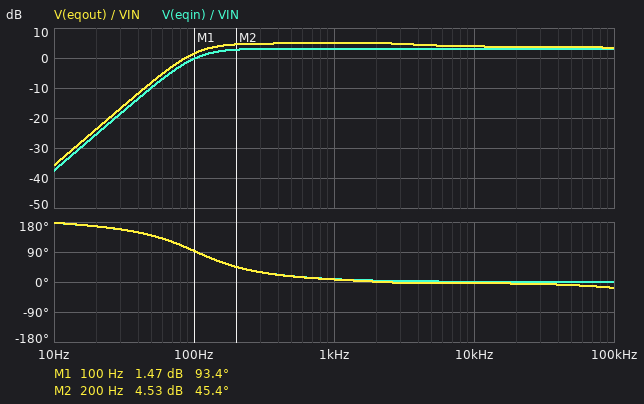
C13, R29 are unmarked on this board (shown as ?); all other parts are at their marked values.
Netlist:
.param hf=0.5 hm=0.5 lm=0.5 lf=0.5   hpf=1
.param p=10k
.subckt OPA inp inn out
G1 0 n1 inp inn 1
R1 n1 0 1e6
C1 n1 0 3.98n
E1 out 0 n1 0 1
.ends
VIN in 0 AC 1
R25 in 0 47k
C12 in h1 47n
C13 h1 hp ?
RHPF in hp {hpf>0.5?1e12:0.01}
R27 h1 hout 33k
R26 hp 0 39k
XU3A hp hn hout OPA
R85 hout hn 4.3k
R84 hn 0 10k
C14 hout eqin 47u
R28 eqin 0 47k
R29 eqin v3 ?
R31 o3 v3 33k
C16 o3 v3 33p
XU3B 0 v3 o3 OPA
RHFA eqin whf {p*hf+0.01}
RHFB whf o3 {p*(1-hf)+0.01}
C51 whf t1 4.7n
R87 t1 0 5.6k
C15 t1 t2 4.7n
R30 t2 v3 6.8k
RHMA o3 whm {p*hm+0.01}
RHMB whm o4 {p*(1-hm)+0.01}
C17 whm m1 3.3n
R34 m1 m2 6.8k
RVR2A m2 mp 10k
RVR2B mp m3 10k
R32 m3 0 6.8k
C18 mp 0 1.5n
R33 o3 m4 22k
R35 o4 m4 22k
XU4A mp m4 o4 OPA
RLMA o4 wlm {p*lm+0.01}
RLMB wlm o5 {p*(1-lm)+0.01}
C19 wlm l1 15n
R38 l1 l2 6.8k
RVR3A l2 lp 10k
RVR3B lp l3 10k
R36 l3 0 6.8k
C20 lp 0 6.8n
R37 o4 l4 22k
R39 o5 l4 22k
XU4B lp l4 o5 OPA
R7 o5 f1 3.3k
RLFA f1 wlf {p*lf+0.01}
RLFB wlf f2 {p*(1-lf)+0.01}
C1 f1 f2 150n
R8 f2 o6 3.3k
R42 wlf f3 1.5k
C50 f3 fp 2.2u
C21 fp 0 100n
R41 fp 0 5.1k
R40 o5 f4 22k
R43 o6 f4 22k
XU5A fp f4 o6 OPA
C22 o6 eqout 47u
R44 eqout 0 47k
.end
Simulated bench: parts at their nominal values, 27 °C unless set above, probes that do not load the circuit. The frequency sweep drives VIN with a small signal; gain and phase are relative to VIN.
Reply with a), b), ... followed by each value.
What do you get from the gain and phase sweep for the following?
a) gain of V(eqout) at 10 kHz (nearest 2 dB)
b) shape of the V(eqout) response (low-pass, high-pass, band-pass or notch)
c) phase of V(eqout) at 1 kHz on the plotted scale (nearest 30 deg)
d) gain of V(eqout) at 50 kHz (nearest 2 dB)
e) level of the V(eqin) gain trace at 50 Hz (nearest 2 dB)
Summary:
a) 4 dB
b) high-pass
c) 0 deg
d) 4 dB
e) -10 dB
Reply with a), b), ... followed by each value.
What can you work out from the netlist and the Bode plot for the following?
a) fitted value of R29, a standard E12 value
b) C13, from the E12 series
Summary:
a) 27 kΩ
b) 39 nF
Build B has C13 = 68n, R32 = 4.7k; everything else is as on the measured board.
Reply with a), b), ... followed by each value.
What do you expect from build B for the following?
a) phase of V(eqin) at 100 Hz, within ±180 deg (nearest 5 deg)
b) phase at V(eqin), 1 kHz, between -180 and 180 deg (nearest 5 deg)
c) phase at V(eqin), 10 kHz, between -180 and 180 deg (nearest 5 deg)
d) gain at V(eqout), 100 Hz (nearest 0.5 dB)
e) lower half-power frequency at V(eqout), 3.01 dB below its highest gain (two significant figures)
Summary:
a) 70 deg
b) 5 deg
c) 0 deg
d) 4.0 dB
e) 74 Hz
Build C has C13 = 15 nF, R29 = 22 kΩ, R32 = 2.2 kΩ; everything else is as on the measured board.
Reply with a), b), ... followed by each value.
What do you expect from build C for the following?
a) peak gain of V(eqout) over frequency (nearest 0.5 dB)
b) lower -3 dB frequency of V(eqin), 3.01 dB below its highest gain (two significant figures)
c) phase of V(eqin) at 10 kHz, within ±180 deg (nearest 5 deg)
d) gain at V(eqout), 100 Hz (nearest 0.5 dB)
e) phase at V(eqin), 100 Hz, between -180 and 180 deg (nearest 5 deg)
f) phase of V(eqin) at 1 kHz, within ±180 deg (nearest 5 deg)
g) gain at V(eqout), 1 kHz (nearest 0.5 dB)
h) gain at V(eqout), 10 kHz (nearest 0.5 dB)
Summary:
a) 7.0 dB
b) 240 Hz
c) 0 deg
d) -4.5 dB
e) 120 deg
f) 20 deg
g) 6.5 dB
h) 5.0 dB
